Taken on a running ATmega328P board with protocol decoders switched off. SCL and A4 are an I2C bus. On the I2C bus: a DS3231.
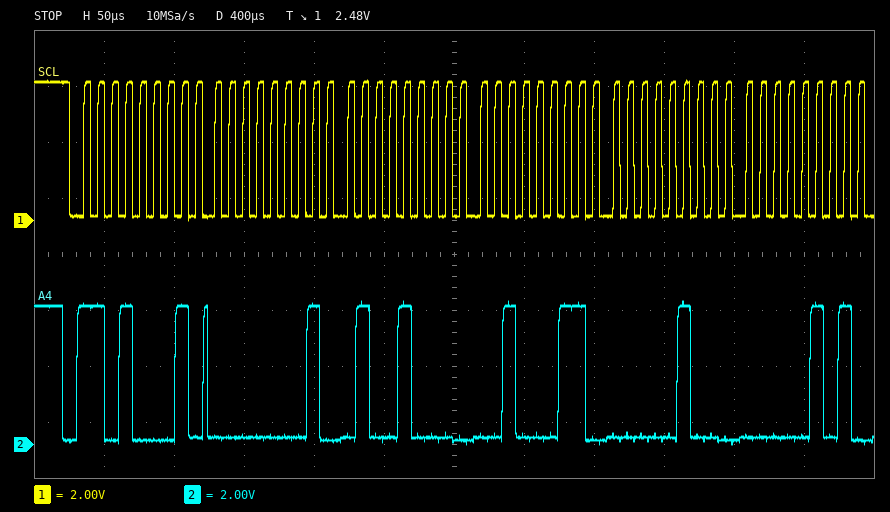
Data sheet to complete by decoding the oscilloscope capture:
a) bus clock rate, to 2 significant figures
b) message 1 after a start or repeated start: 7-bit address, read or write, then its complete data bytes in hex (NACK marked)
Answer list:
100 kHz
0x68 read: 01 48 23 04 05
